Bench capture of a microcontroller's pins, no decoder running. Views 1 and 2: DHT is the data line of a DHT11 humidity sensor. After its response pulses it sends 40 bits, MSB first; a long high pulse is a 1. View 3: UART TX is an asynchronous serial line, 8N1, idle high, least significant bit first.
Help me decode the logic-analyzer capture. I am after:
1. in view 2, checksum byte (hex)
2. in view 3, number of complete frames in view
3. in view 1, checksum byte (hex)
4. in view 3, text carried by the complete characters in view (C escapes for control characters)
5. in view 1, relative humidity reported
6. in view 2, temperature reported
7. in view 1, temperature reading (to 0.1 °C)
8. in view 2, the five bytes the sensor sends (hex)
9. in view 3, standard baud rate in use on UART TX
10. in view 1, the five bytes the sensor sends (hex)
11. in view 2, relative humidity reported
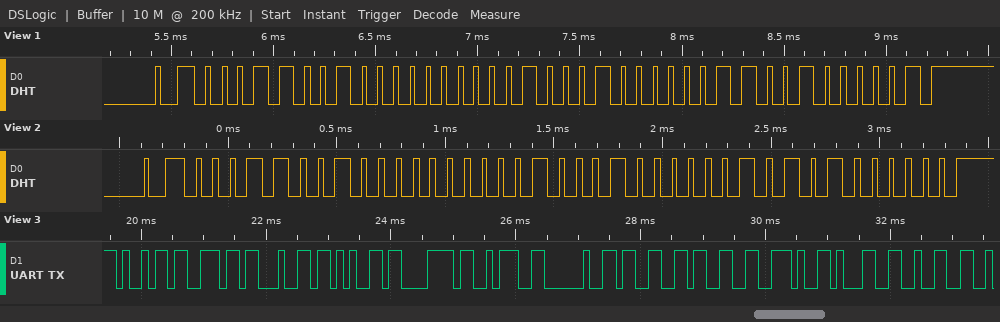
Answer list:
0x40
12
0x41
"index: 33.12"
25 %
34.5 °C
34.6 °C
19 00 22 05 40
9600 baud
19 00 22 06 41
25 %
